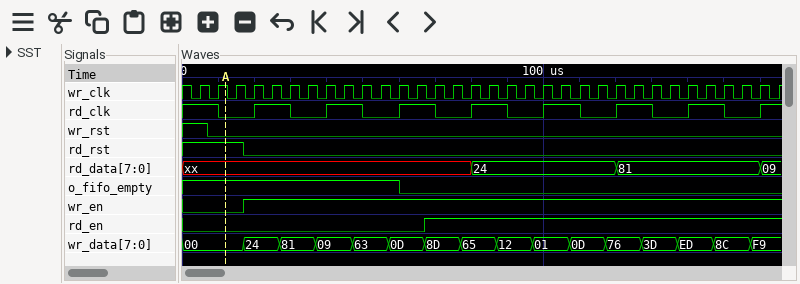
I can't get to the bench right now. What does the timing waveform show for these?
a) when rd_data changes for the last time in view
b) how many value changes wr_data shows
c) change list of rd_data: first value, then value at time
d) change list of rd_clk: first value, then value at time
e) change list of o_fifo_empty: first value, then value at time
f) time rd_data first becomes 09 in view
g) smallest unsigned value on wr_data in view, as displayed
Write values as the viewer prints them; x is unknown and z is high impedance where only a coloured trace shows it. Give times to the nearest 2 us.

160 us
15
xx, 24 at 80 us, 81 at 120 us, 09 at 160 us
1, 0 at 10 us, 1 at 20 us, 0 at 30 us, 1 at 40 us, 0 at 50 us, 1 at 60 us, 0 at 70 us, 1 at 80 us, 0 at 90 us, 1 at 100 us, 0 at 110 us, 1 at 120 us, 0 at 130 us, 1 at 140 us, 0 at 150 us, 1 at 160 us
1, 0 at 60 us
160 us
00
